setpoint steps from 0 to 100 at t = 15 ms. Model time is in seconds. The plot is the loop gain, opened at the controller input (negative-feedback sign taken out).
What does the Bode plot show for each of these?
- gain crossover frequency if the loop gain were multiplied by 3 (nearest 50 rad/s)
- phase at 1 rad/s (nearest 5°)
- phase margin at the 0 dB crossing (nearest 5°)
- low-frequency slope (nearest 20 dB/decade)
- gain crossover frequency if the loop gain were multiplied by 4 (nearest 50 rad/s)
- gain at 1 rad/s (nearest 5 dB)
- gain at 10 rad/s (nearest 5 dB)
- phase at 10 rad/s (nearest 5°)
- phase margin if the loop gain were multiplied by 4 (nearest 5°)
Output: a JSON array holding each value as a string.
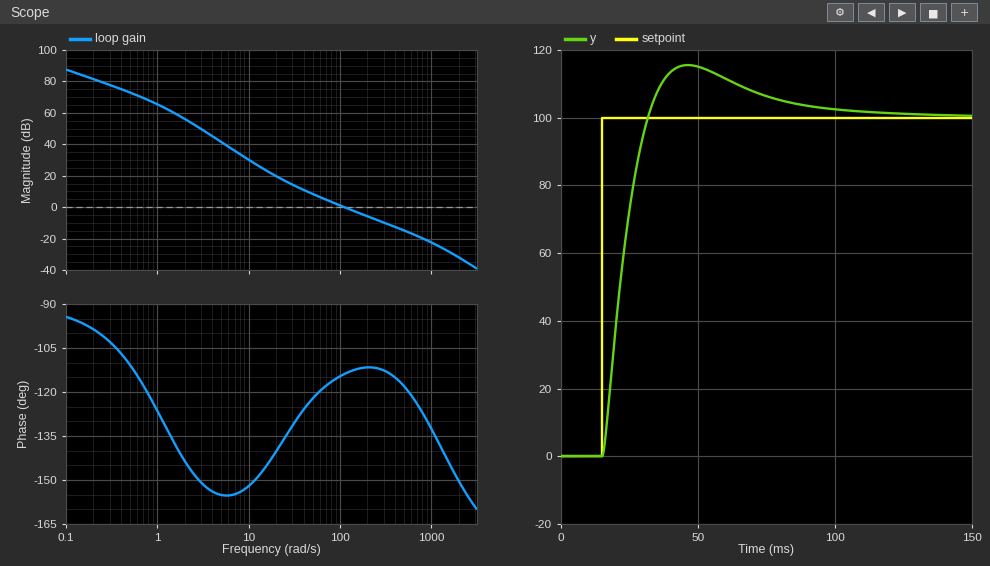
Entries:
["300 rad/s", "-125°", "65°", "-20 dB/decade", "400 rad/s", "65 dB", "30 dB", "-150°", "65°"]
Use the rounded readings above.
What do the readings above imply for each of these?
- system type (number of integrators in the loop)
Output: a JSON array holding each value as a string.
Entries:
["1"]
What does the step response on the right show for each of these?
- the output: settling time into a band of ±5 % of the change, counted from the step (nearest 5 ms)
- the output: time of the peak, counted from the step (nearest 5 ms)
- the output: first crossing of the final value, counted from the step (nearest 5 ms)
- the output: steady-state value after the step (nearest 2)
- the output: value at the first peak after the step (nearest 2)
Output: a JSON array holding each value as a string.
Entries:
["65 ms", "30 ms", "15 ms", "100", "116"]
